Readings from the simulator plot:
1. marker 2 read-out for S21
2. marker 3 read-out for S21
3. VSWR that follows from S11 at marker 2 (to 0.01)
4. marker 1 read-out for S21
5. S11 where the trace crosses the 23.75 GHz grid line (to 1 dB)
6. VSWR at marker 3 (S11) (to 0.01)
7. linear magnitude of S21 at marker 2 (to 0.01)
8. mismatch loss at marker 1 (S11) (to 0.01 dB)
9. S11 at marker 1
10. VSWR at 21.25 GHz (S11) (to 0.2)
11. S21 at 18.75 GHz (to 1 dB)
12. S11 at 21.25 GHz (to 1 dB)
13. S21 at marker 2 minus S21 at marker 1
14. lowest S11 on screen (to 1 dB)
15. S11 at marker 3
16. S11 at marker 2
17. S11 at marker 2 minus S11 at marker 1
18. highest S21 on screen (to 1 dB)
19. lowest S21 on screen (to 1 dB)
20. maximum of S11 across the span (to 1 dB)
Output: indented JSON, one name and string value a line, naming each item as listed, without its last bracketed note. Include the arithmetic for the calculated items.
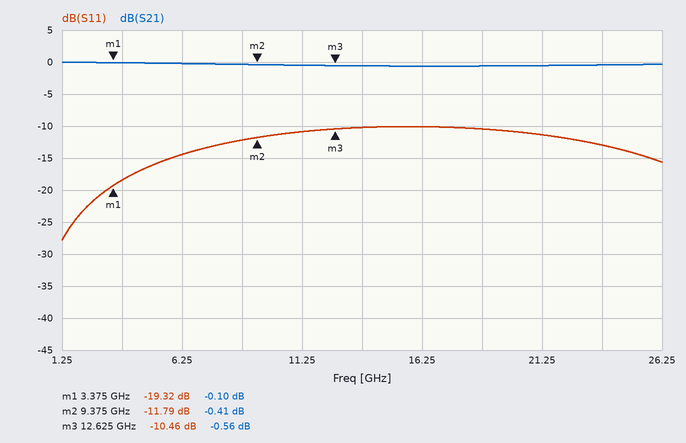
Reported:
{
  "marker 2 read-out for S21": "-0.41 dB",
  "marker 3 read-out for S21": "-0.56 dB",
  "VSWR that follows from S11 at marker 2": "(1 + 0.2573)/(1 − 0.2573) ≈ 1.69",
  "marker 1 read-out for S21": "-0.10 dB",
  "S11 where the trace crosses the 23.75 GHz grid line": "-13 dB",
  "VSWR at marker 3 (S11)": "(1 + 0.2999)/(1 − 0.2999) ≈ 1.86",
  "linear magnitude of S21 at marker 2": "10^(-0.41/20) ≈ 0.95",
  "mismatch loss at marker 1 (S11)": "−10 log10(1 − 10^(-19.32/10)) ≈ 0.05 dB",
  "S11 at marker 1": "-19.32 dB",
  "VSWR at 21.25 GHz (S11)": "|Γ| = 10^(-11/20) = 0.2818; VSWR = (1 + 0.2818)/(1 − 0.2818) ≈ 1.8",
  "S21 at 18.75 GHz": "-1 dB",
  "S11 at 21.25 GHz": "-11 dB",
  "S21 at marker 2 minus S21 at marker 1": "-0.41 − (-0.1) = -0.31 dB",
  "lowest S11 on screen": "-28 dB",
  "S11 at marker 3": "-10.46 dB",
  "S11 at marker 2": "-11.79 dB",
  "S11 at marker 2 minus S11 at marker 1": "-11.79 − (-19.32) = 7.53 dB",
  "highest S21 on screen": "0 dB",
  "lowest S21 on screen": "-1 dB",
  "maximum of S11 across the span": "-10 dB"
}
